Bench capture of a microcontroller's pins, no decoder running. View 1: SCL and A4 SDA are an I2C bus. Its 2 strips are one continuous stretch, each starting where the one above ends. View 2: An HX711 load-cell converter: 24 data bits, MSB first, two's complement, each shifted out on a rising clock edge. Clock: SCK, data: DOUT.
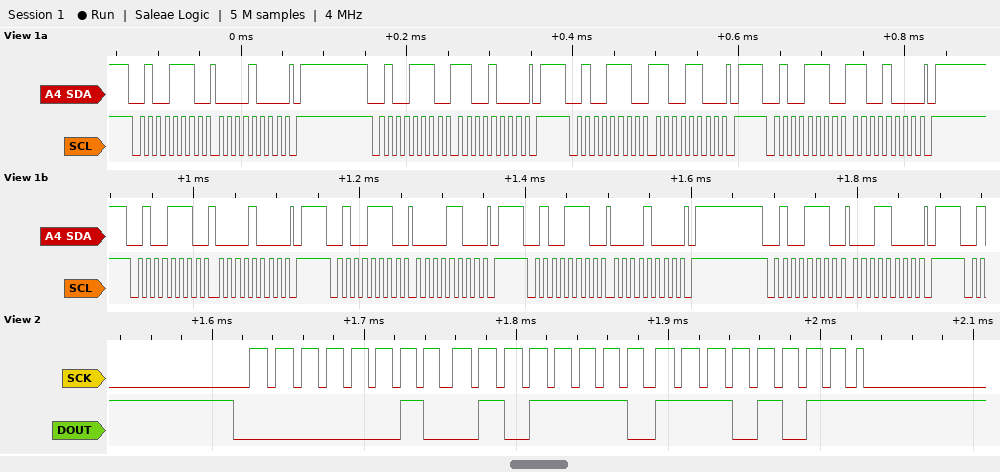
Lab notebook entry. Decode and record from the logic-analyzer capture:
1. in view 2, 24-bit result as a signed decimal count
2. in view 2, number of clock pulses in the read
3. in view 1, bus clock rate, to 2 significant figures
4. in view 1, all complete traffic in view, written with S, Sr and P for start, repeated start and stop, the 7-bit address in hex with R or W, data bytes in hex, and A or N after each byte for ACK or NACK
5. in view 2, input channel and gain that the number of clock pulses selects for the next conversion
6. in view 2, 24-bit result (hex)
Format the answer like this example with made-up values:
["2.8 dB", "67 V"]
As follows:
["155371", "25", "100 kHz", "S 27W A 08 A P S 27W A C8 A P S 27W A CC A P S 27W A C8 A P S 27W A 08 A P S 27W A 0C A P S 27W A 08 A P S 27W A 18 A P", "channel A, gain 128", "0x025EEB"]
